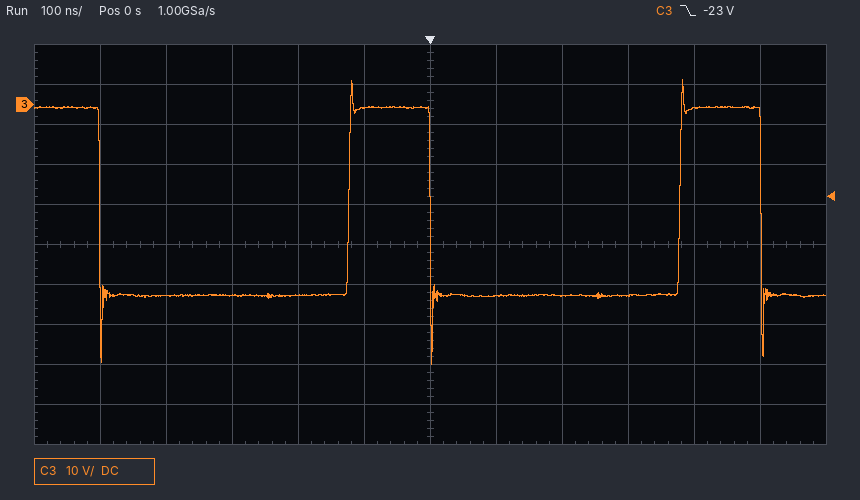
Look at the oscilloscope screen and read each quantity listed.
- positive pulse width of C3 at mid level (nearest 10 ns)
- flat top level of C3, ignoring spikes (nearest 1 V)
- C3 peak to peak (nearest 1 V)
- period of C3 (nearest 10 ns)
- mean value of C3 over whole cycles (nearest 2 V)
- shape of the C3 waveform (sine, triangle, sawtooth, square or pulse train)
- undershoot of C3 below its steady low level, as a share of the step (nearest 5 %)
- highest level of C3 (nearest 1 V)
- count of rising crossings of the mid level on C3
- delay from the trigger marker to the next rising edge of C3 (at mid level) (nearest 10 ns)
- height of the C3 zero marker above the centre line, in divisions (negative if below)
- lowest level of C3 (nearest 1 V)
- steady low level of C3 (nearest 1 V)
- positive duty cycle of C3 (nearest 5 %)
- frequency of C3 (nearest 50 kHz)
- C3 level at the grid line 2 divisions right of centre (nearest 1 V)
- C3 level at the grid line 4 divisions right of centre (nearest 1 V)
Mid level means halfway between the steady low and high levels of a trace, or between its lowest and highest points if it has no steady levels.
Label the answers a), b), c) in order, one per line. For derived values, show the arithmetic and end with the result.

a) 120 ns
b) -1 V
c) 6 V − (-65 V) = 71 V
d) 500 ns
e) -48 V + 0.25 × (-1 V − (-48 V)) ≈ -36 V
f) pulse train
g) 35 %
h) 6 V
i) 2
j) 380 ns
k) +3.5 div
l) -65 V
m) -48 V
n) 120 ns / 500 ns ≈ 24.0 %, so 25 % to the nearest 5 %
o) 1 / 500 ns ≈ 2.00 MHz
p) -48 V
q) -1 V
